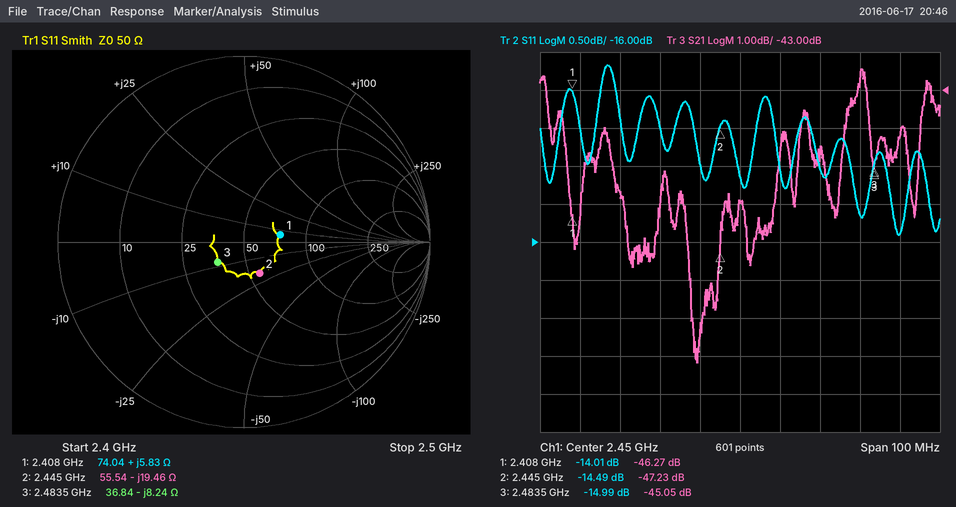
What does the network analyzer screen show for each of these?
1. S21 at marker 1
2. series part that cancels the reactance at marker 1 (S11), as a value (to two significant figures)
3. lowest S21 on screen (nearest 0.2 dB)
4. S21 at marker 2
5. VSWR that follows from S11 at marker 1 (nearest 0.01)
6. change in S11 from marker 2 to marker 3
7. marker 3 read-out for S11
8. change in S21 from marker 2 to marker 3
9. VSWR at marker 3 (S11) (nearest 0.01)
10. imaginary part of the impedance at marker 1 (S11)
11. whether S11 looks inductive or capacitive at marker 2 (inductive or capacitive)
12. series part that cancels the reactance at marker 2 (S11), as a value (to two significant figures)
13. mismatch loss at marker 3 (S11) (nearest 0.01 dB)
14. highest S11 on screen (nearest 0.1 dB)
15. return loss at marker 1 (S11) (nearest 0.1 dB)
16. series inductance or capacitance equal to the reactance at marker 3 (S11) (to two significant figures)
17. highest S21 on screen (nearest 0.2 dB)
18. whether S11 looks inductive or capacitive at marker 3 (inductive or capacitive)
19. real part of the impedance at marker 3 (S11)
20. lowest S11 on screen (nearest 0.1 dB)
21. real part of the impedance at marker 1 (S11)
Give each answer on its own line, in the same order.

-46.27 dB
11 pF
-50.2 dB
-47.23 dB
1.50
-0.50 dB
-14.99 dB
2.18 dB
1.43
+5.83 Ω
capacitive
1.3 nH
0.14 dB
-13.7 dB
14.0 dB
7.8 pF
-42.4 dB
capacitive
36.84 Ω
-15.9 dB
74.04 Ω
